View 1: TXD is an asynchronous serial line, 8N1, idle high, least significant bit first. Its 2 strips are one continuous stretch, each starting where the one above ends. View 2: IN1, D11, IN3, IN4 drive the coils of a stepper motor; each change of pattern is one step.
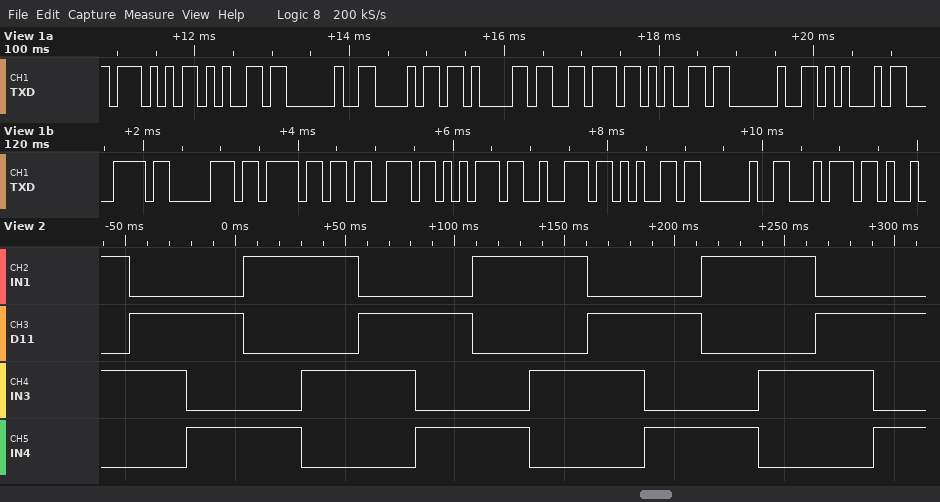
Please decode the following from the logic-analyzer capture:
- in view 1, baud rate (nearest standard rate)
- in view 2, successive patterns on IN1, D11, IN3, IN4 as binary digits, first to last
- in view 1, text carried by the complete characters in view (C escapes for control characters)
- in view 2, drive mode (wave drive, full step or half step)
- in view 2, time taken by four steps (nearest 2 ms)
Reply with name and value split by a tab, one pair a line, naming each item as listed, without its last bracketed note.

in view 1, baud rate	9600 baud
in view 2, successive patterns on IN1, D11, IN3, IN4 as binary digits, first to last	1010 0110 0101 1001 1010 0110 0101 1001 1010 0110 0101 1001 1010 0110 0101
in view 1, text carried by the complete characters in view	"We have Exposure t"
in view 2, drive mode	full step
in view 2, time taken by four steps	104 ms
